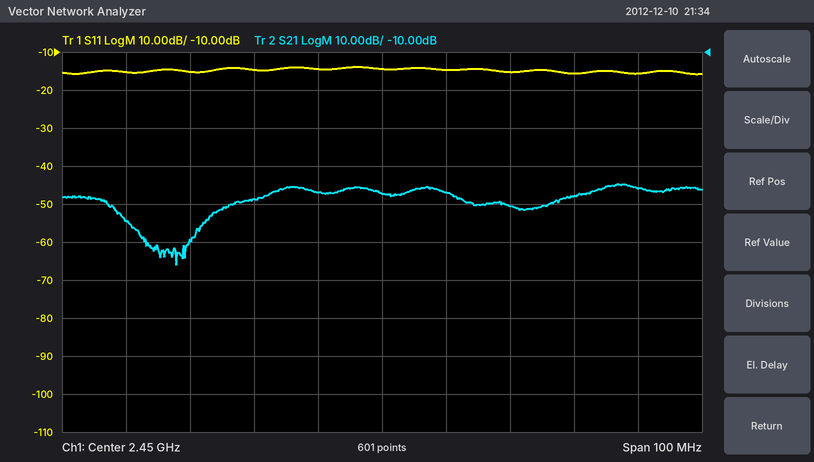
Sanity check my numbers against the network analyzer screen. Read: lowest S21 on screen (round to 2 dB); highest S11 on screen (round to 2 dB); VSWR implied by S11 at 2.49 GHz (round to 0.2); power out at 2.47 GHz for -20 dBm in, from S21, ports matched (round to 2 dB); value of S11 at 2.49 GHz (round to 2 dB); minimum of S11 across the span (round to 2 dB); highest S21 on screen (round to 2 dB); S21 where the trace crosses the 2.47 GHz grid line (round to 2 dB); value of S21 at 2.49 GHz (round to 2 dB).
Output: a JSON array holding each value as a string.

["-66 dB", "-14 dB", "1.4", "-70 dBm", "-16 dB", "-16 dB", "-44 dB", "-50 dB", "-46 dB"]
